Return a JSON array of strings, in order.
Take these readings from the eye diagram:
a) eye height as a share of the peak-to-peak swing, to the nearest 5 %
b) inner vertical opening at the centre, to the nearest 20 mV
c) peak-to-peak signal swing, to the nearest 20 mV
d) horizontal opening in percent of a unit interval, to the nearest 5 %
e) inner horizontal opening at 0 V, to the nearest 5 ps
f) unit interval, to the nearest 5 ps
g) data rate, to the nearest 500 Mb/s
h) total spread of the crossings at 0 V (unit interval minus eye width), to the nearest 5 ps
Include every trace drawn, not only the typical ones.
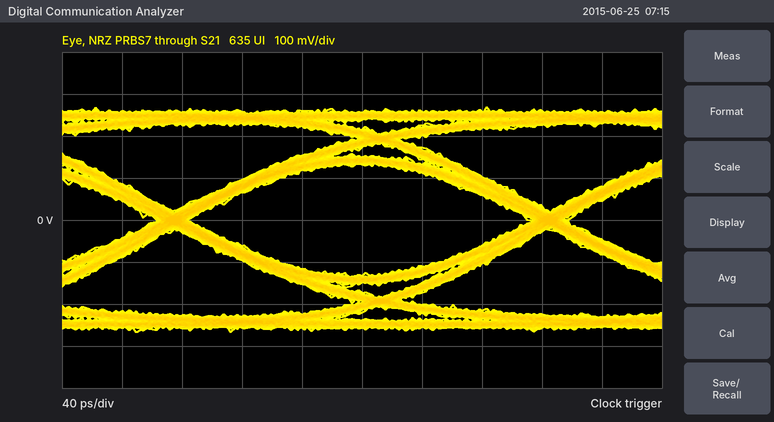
["50 %", "260 mV", "540 mV", "90 %", "225 ps", "250 ps", "4.0 Gb/s", "25 ps"]
